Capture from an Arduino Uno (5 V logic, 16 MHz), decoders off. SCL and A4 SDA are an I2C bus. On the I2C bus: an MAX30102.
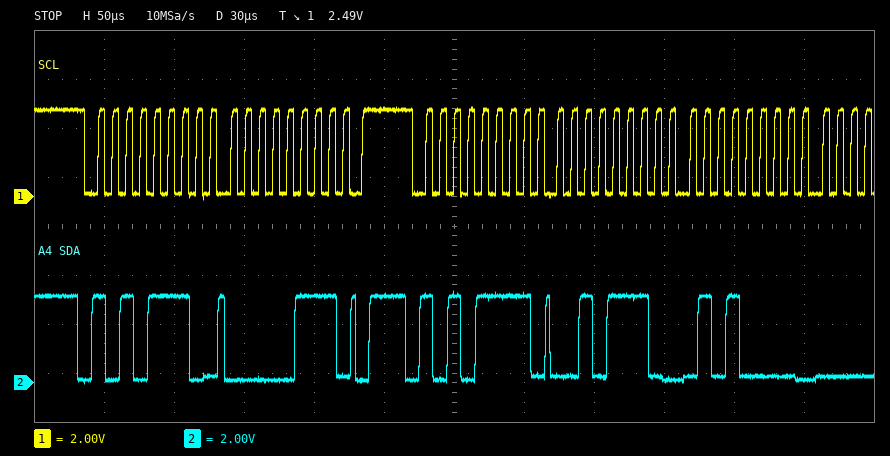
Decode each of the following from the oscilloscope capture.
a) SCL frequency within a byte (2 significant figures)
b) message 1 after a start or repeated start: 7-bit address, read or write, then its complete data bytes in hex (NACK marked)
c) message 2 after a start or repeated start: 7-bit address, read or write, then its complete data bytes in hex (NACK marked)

100 kHz
0x57 write: 07
0x57 read: 2E 50
